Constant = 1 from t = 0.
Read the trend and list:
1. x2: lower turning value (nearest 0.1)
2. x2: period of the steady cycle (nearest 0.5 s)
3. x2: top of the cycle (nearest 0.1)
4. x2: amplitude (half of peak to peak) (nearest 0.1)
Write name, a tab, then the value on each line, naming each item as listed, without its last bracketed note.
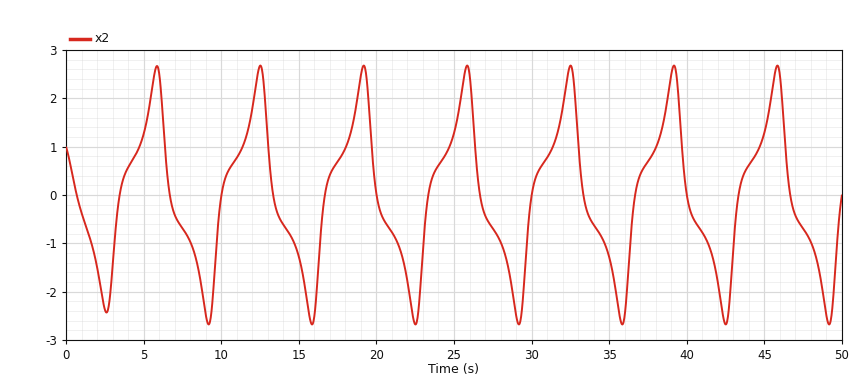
x2: lower turning value	-2.7
x2: period of the steady cycle	6.5 s
x2: top of the cycle	2.7
x2: amplitude (half of peak to peak)	2.7
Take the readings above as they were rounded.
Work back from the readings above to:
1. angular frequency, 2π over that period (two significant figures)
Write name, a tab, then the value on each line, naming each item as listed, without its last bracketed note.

angular frequency, 2π over that period	0.97 rad/s
